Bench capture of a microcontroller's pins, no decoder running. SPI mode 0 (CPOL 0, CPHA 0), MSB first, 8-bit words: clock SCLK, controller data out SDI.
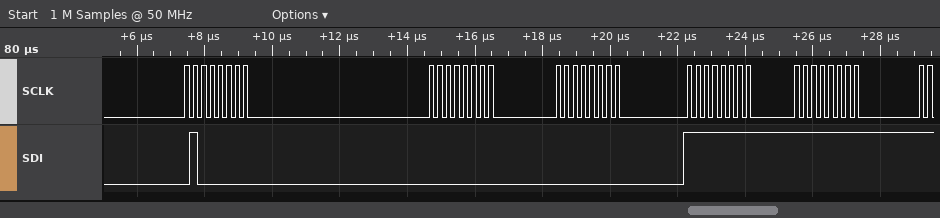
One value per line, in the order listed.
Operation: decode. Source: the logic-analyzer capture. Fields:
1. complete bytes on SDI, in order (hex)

40 00 00 FF FF
